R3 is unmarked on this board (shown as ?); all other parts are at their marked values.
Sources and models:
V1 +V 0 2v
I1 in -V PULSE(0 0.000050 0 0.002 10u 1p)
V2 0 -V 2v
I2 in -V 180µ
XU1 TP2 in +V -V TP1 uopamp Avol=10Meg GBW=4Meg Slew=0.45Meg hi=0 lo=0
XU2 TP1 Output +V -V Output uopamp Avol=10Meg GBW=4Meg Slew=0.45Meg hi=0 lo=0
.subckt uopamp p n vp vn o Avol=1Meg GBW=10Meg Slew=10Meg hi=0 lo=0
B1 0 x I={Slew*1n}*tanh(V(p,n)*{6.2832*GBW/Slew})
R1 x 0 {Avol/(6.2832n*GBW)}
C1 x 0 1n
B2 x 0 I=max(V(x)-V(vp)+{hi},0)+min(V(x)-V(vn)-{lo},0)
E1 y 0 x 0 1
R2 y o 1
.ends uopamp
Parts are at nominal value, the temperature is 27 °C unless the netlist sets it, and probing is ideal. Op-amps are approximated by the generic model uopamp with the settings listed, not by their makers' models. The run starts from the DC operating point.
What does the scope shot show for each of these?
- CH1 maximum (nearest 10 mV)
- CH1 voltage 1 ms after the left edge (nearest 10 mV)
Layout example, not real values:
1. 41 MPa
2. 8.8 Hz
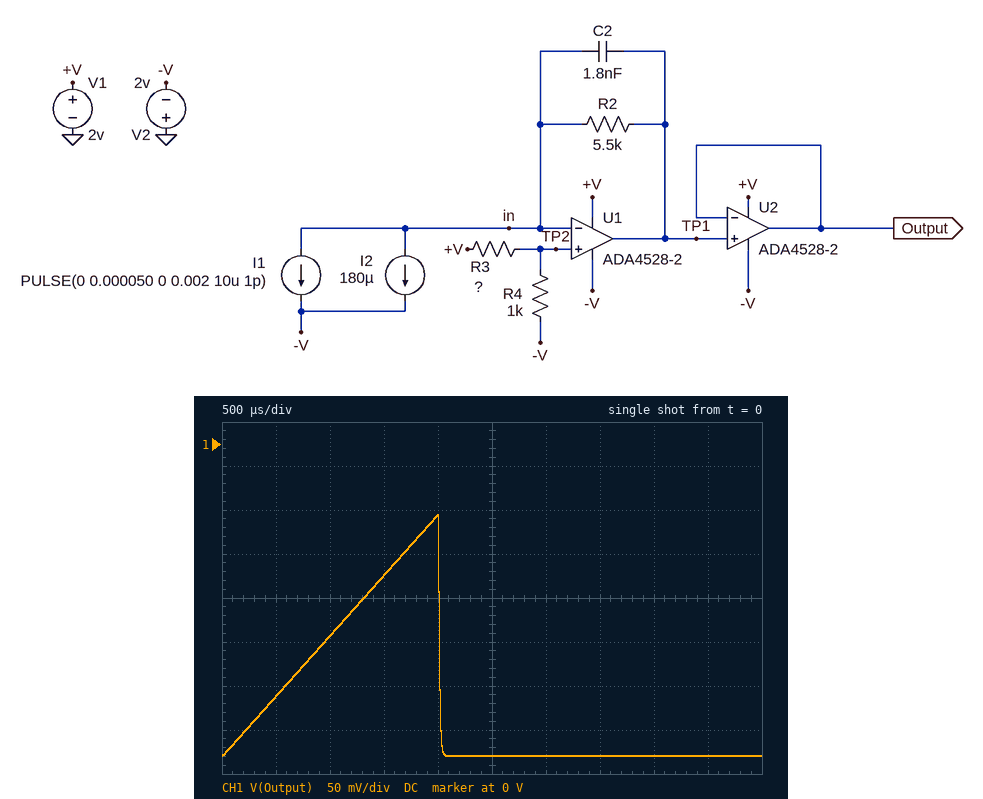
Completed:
1. -80 mV
2. -220 mV
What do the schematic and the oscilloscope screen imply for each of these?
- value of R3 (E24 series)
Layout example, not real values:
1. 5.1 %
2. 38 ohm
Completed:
1. 5.1 kΩ
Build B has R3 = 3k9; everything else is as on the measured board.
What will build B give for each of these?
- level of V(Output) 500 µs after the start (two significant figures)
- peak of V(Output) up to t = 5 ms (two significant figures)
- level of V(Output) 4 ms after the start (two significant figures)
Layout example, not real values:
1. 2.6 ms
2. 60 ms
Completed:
1. -130 mV
2. 80 mV
3. -190 mV
